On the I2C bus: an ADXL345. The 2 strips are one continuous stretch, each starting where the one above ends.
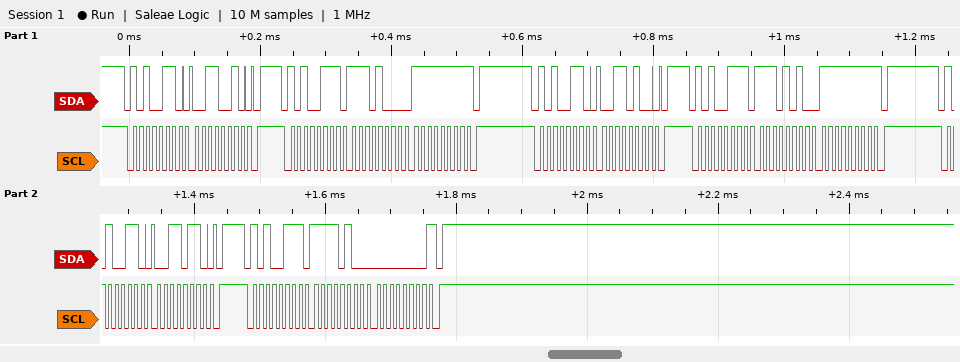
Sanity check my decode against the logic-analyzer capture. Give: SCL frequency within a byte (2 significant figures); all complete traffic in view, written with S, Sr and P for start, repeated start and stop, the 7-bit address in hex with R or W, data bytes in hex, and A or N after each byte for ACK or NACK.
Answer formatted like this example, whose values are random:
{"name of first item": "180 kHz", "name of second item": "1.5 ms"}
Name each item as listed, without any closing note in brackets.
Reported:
{"SCL frequency within a byte": "100 kHz", "all complete traffic in view, written with S, Sr and P for start, repeated start and stop, the 7-bit address in hex with R or W, data bytes in hex, and A or N after each byte for ACK or NACK": "S 53W A 32 A P S 53R A E8 A FF N P S 53W A 34 A P S 53R A EA A FF N P S 53W A 36 A P S 53R A F4 A 00 N P"}
